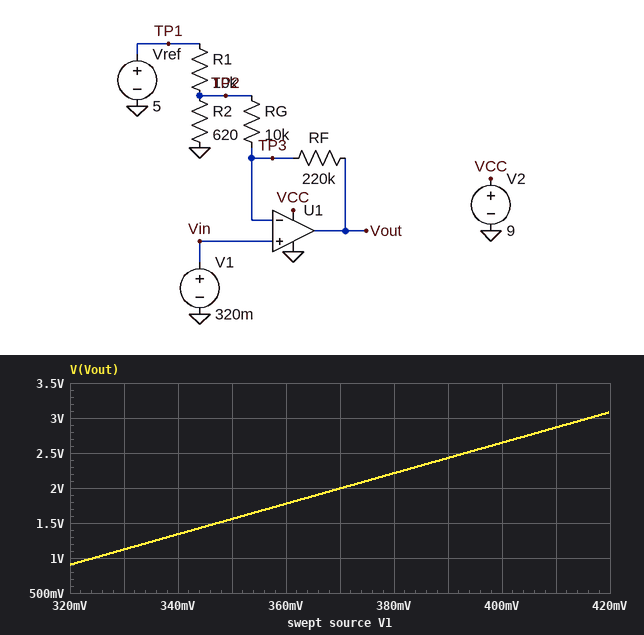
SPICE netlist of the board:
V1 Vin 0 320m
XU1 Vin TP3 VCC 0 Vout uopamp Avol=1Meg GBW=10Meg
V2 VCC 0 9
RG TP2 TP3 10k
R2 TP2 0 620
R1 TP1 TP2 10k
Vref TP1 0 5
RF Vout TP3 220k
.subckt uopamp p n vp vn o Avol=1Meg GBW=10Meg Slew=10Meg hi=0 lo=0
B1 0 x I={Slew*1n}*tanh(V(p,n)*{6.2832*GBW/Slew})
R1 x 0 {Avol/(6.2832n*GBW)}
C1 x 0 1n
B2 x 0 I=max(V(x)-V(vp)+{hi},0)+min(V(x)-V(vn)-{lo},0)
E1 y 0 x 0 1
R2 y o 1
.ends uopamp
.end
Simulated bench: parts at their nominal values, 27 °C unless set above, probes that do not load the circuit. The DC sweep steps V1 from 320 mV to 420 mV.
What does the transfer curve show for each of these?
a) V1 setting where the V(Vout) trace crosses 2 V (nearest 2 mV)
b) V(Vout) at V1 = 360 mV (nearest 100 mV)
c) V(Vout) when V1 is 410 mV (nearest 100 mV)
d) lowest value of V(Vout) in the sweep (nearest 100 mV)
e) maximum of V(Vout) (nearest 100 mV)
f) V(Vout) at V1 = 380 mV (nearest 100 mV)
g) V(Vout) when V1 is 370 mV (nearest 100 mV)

370 mV
1.8 V
2.9 V
900 mV
3.1 V
2.2 V
2.0 V
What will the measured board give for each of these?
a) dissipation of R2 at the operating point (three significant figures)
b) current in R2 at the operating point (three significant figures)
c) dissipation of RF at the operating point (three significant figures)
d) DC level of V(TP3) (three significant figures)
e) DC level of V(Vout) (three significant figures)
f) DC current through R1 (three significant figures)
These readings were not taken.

139 µW
473 µA
1.55 µW
320 mV
904 mV
471 µA
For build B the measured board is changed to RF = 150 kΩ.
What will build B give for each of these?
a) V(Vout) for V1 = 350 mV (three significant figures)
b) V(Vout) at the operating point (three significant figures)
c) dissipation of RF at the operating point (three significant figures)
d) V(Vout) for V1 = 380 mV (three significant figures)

1.17 V
718 mV
1.06 µW
1.63 V
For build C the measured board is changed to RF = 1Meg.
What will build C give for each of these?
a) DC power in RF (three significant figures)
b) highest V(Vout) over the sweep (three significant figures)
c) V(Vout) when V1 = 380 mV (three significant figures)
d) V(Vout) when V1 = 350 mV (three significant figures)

7.05 µW
9.00 V
8.70 V
5.84 V
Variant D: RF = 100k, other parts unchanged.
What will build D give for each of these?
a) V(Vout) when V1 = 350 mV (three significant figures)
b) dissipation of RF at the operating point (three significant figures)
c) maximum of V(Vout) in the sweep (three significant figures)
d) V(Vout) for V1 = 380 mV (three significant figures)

899 mV
705 nW
1.63 V
1.21 V
